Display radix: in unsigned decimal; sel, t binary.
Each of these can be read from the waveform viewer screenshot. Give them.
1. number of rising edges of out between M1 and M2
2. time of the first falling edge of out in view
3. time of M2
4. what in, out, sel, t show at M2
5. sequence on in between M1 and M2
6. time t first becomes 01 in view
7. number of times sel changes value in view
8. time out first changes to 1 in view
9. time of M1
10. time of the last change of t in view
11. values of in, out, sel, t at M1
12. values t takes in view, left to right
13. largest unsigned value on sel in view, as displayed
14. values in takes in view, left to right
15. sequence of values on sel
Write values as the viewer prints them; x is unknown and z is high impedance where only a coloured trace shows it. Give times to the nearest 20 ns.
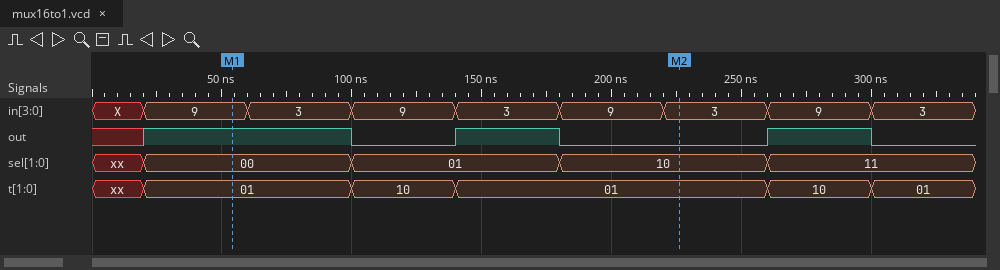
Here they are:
1
100 ns
220 ns
in=3, out=0, sel=10, t=01
9, 3, 9, 3, 9, 3
20 ns
4
20 ns
60 ns
300 ns
in=9, out=1, sel=00, t=01
xx, 01, 10, 01, 10, 01
11
X, 9, 3, 9, 3, 9, 3, 9, 3
xx, 00, 01, 10, 11
